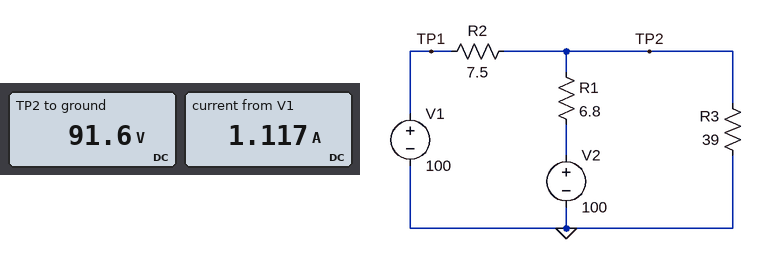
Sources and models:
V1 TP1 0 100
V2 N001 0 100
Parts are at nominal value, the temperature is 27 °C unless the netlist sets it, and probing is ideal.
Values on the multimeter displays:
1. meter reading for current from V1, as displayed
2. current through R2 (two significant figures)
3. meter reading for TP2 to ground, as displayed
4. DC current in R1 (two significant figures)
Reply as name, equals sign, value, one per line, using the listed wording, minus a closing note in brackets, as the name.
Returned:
meter reading for current from V1, as displayed = 1.117 A
current through R2 = 1.1 A
meter reading for TP2 to ground, as displayed = 91.6 V
DC current in R1 = 1.2 A
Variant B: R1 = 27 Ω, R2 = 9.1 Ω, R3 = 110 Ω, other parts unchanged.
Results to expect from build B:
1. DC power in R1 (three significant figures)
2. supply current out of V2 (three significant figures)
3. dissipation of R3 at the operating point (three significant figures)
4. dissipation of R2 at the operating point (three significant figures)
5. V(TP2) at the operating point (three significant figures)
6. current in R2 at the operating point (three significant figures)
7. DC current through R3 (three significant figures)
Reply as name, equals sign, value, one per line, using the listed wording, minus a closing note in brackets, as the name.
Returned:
DC power in R1 = 1.26 W
supply current out of V2 = 216 mA
dissipation of R3 at the operating point = 80.6 W
dissipation of R2 at the operating point = 3.73 W
V(TP2) at the operating point = 94.2 V
current in R2 at the operating point = 640 mA
DC current through R3 = 856 mA
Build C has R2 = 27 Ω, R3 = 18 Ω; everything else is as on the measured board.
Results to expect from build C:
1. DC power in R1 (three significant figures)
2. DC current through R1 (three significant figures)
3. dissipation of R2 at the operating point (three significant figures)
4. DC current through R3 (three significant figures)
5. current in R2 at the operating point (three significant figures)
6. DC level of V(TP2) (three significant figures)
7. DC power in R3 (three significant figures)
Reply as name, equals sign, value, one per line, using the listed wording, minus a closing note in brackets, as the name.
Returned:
DC power in R1 = 79.0 W
DC current through R1 = 3.41 A
dissipation of R2 at the operating point = 19.9 W
DC current through R3 = 4.27 A
current in R2 at the operating point = 859 mA
DC level of V(TP2) = 76.8 V
DC power in R3 = 328 W
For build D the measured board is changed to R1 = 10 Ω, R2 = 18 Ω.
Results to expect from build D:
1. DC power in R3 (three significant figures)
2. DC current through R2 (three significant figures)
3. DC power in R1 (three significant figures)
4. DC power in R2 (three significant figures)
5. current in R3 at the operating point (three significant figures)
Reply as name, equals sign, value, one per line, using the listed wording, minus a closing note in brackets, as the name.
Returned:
DC power in R3 = 189 W
DC current through R2 = 786 mA
DC power in R1 = 20.0 W
DC power in R2 = 11.1 W
current in R3 at the operating point = 2.20 A
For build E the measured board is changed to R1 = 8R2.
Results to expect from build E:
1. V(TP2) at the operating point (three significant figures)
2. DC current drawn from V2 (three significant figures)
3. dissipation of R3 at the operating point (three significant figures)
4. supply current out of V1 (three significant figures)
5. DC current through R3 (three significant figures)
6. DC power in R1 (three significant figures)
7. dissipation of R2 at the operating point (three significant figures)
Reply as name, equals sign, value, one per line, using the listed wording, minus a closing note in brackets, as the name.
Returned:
V(TP2) at the operating point = 90.9 V
DC current drawn from V2 = 1.11 A
dissipation of R3 at the operating point = 212 W
supply current out of V1 = 1.22 A
DC current through R3 = 2.33 A
DC power in R1 = 10.2 W
dissipation of R2 at the operating point = 11.1 W
